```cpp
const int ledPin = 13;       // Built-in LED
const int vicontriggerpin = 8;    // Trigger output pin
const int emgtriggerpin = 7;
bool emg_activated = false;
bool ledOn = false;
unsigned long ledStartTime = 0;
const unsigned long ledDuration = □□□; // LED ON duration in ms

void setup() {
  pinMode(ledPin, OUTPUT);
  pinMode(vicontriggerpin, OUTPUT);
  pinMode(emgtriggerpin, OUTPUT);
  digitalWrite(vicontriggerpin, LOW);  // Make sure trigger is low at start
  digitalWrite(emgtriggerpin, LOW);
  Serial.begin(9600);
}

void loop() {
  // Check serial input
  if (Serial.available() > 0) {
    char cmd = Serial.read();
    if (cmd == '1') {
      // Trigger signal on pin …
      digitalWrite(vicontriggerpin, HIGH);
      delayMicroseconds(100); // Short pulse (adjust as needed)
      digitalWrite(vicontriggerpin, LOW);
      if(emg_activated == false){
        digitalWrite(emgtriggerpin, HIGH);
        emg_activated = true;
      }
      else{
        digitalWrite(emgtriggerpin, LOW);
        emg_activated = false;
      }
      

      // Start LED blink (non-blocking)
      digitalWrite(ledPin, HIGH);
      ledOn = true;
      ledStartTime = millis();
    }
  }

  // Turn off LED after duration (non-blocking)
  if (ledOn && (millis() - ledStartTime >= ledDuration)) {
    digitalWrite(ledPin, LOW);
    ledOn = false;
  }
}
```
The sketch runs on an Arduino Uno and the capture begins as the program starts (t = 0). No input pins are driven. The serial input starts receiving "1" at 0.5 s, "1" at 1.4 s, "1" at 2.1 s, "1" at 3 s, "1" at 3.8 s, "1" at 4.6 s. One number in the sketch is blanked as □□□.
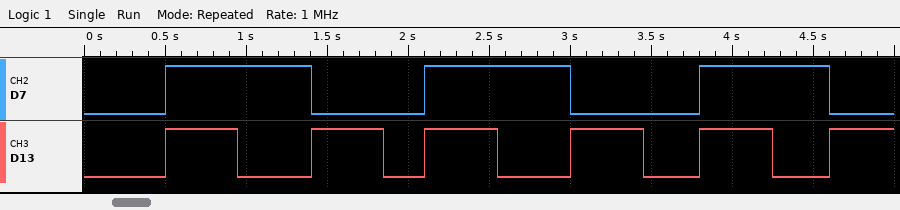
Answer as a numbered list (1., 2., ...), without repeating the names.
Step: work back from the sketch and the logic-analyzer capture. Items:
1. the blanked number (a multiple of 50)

1. 450
